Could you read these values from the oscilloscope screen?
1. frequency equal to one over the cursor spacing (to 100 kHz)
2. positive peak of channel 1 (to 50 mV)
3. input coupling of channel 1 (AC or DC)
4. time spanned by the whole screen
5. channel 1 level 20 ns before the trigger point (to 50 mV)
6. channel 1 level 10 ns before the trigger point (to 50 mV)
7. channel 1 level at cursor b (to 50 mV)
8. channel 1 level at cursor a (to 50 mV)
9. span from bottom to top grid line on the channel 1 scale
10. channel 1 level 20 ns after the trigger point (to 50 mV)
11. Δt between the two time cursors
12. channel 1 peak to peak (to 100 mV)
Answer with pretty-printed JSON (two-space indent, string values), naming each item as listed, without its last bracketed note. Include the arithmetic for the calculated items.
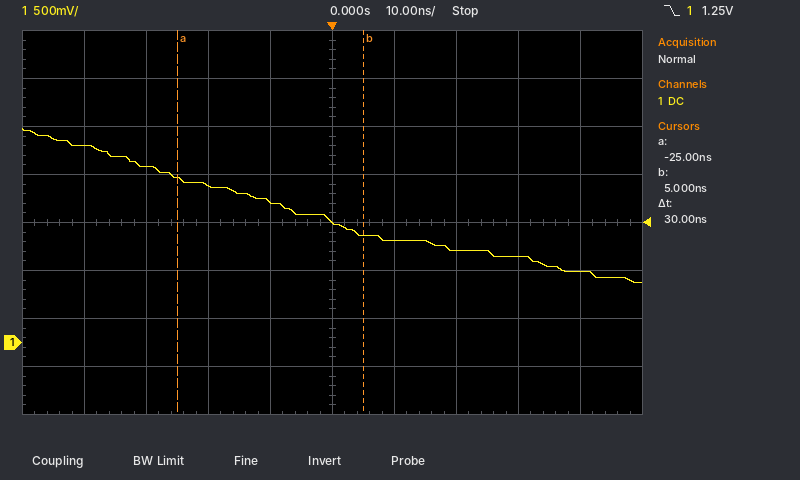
{
  "frequency equal to one over the cursor spacing": "1 / 30 ns ≈ 33.3 MHz",
  "positive peak of channel 1": "2.25 V",
  "input coupling of channel 1": "DC",
  "time spanned by the whole screen": "100 ns",
  "channel 1 level 20 ns before the trigger point": "1.65 V",
  "channel 1 level 10 ns before the trigger point": "1.45 V",
  "channel 1 level at cursor b": "1.10 V",
  "channel 1 level at cursor a": "1.70 V",
  "span from bottom to top grid line on the channel 1 scale": "4 V",
  "channel 1 level 20 ns after the trigger point": "950 mV",
  "Δt between the two time cursors": "30 ns",
  "channel 1 peak to peak": "1.60 V"
}
